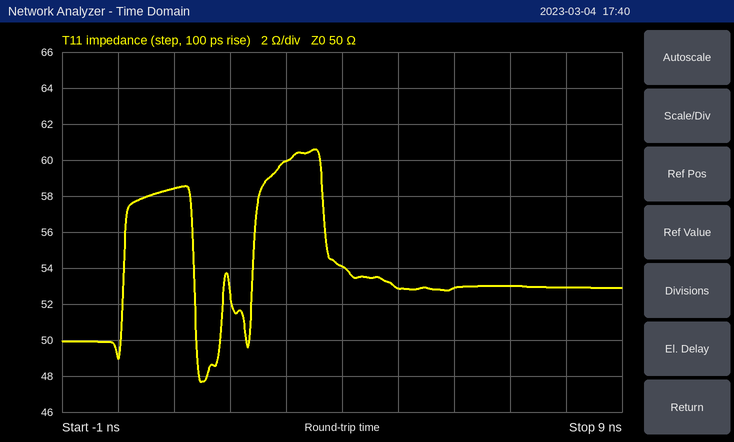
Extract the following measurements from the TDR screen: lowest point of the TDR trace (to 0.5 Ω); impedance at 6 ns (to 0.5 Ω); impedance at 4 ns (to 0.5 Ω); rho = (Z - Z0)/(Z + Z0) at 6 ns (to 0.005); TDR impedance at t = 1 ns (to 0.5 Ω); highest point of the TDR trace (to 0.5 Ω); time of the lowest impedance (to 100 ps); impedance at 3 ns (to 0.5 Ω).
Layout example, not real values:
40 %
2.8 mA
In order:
47.5 Ω
53.0 Ω
54.0 Ω
+0.030
58.5 Ω
60.5 Ω
1.5 ns
60.0 Ω
